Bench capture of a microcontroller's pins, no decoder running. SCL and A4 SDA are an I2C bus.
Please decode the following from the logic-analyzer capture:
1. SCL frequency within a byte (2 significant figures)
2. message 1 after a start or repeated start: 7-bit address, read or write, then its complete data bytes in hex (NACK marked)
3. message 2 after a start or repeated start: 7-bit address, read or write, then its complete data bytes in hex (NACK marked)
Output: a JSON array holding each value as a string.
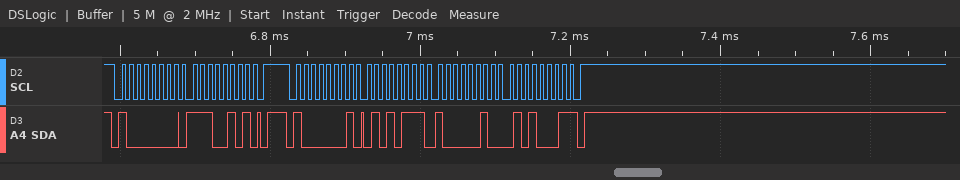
["100 kHz", "0x40 write: E5", "0x40 read: 57 82 51 NACK"]
